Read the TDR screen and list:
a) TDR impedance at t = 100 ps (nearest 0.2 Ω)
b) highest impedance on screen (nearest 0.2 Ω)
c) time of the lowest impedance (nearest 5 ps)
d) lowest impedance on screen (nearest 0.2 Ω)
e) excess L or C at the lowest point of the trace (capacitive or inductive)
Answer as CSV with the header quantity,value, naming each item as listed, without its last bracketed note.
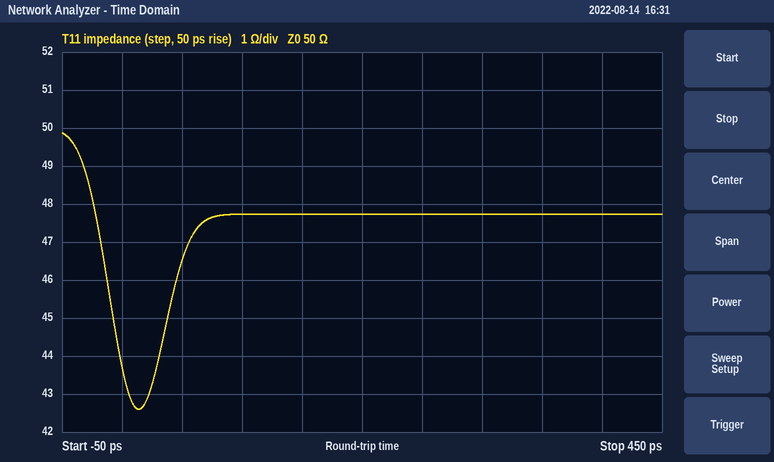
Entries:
quantity,value
TDR impedance at t = 100 ps,47.8 Ω
highest impedance on screen,49.8 Ω
time of the lowest impedance,15 ps
lowest impedance on screen,42.6 Ω
excess L or C at the lowest point of the trace,capacitive
